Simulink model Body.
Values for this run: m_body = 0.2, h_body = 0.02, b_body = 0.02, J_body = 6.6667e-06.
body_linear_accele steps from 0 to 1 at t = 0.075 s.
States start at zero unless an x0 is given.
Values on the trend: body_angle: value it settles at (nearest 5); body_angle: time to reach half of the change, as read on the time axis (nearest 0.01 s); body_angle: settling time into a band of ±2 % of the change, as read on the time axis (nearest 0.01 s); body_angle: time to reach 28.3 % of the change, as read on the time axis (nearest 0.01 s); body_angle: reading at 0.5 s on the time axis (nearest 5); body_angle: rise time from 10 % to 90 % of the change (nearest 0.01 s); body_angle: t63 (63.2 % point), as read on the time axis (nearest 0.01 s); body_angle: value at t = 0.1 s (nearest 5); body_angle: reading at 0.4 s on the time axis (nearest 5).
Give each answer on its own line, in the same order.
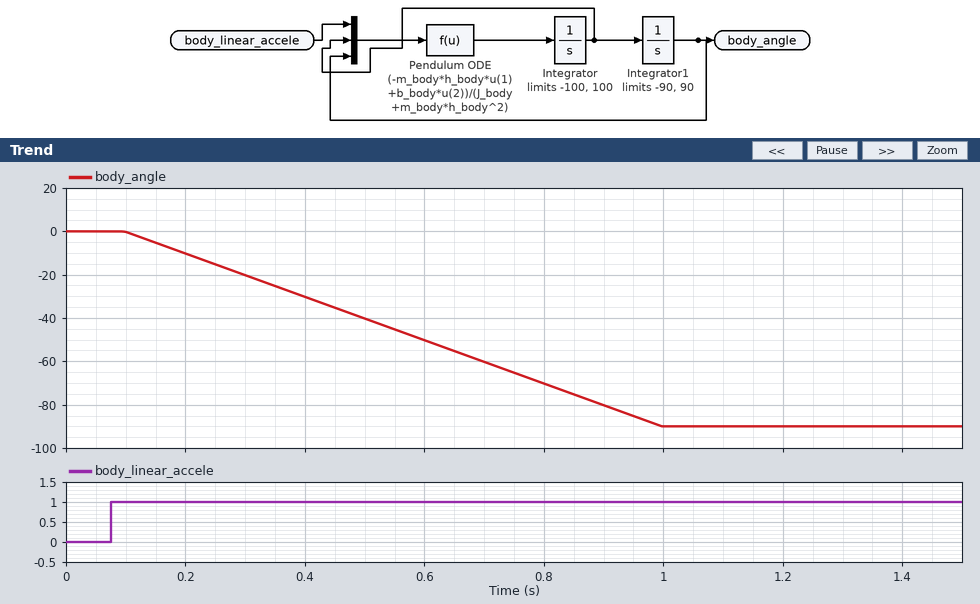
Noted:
-90
0.55 s
0.98 s
0.35 s
-40
0.72 s
0.67 s
0
-30
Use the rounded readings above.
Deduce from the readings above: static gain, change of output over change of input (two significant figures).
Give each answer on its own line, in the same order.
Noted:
-90
